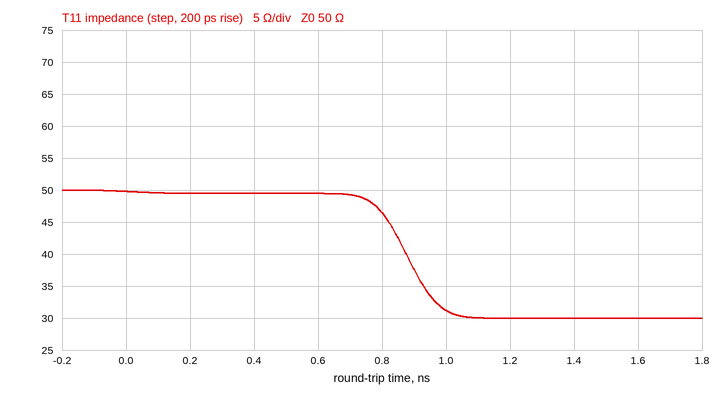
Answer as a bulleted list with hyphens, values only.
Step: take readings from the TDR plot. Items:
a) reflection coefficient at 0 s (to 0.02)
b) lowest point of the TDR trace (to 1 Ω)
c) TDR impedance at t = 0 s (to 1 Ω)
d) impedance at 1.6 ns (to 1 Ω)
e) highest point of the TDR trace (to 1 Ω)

- 0.00
- 30 Ω
- 50 Ω
- 30 Ω
- 50 Ω
